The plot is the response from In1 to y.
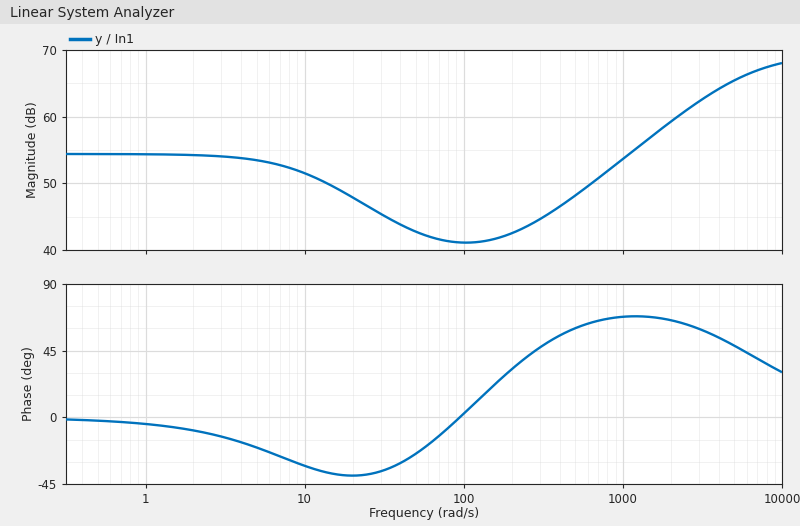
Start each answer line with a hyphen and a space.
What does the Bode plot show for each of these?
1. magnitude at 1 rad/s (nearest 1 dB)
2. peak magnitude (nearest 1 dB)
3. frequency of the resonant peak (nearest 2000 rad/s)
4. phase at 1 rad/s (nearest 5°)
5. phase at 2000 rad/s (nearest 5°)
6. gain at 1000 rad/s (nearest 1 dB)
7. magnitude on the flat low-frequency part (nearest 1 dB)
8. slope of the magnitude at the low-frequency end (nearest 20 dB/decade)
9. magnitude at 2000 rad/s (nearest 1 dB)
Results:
- 54 dB
- 68 dB
- 10000 rad/s
- -5°
- 65°
- 54 dB
- 54 dB
- 0 dB/decade
- 59 dB
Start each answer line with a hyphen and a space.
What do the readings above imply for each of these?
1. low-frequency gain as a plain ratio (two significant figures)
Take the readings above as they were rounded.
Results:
- 500
